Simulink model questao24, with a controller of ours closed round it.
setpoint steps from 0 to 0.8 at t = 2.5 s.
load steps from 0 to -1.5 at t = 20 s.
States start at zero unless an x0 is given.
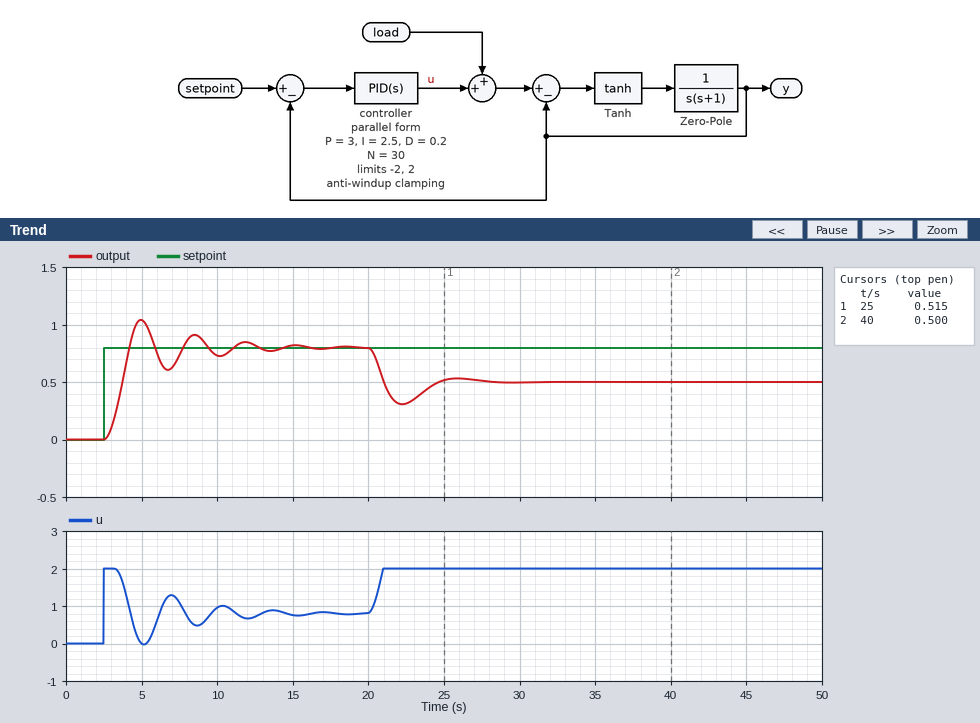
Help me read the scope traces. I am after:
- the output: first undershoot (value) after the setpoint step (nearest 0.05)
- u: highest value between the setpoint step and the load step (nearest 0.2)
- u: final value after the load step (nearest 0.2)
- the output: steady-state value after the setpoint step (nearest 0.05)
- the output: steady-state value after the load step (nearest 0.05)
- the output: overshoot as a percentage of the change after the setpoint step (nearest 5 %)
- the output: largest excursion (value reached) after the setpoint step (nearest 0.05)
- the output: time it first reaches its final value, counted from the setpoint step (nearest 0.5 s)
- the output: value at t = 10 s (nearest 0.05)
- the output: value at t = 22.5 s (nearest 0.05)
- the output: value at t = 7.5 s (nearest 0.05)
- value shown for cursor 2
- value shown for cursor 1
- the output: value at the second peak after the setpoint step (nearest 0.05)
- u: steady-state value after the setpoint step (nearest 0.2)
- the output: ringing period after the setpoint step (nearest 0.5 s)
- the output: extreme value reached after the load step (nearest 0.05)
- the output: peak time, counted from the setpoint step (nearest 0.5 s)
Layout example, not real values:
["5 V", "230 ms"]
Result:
["0.60", "2.0", "2.0", "0.80", "0.50", "30 %", "1.05", "1.5 s", "0.75", "0.30", "0.75", "0.500", "0.515", "0.90", "0.8", "3.5 s", "0.30", "2.5 s"]
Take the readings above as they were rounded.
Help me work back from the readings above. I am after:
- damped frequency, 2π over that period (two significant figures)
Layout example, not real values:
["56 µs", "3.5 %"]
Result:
["1.8 rad/s"]
